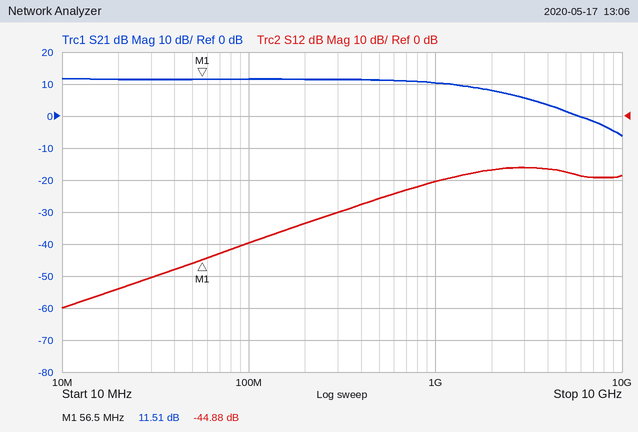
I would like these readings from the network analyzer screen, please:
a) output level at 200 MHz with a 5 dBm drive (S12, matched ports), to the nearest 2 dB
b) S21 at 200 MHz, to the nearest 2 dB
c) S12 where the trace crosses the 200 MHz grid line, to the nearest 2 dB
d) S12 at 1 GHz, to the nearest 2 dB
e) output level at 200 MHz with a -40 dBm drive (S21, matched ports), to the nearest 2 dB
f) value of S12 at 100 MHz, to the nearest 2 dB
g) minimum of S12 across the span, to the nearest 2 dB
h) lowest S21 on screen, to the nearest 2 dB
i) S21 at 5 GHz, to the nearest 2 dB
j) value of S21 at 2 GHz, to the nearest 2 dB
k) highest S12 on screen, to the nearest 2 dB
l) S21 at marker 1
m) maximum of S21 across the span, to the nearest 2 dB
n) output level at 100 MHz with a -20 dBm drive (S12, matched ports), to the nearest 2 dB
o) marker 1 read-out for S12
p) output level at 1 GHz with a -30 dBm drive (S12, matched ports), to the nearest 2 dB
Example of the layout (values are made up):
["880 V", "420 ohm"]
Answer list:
["-28 dBm", "12 dB", "-34 dB", "-20 dB", "-28 dBm", "-40 dB", "-60 dB", "-6 dB", "2 dB", "8 dB", "-16 dB", "11.51 dB", "12 dB", "-60 dBm", "-44.88 dB", "-50 dBm"]
